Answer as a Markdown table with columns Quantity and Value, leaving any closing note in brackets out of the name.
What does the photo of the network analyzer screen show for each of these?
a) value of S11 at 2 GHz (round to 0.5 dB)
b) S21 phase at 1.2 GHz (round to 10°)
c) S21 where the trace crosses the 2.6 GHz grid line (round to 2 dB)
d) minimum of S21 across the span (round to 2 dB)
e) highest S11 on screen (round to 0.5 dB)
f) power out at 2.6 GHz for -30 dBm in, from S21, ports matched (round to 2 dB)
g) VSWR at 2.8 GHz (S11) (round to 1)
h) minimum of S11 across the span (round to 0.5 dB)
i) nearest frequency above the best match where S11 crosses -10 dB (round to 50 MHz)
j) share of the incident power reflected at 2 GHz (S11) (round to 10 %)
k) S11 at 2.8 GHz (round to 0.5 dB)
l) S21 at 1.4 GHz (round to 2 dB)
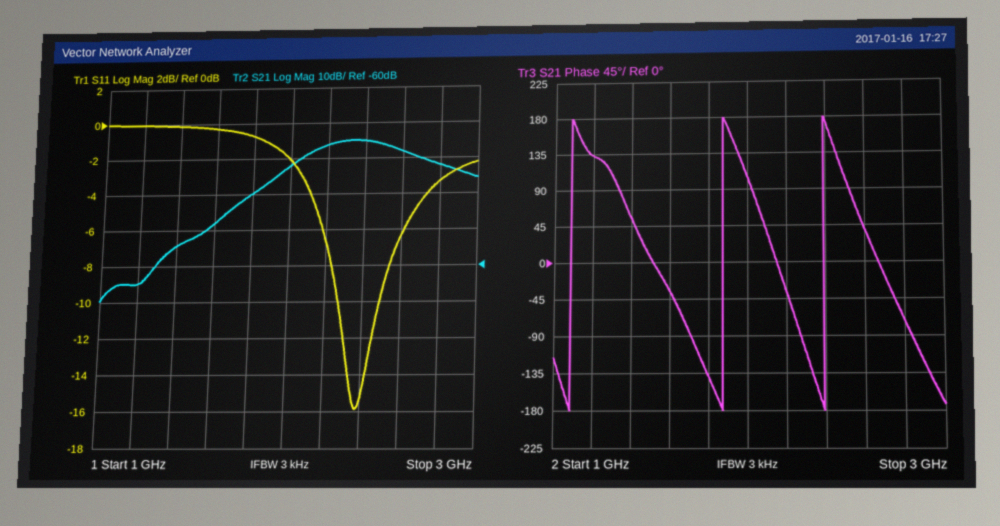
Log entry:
| Quantity | Value |
|---|---|
| value of S11 at 2 GHz | -2.0 dB |
| S21 phase at 1.2 GHz | 130° |
| S21 where the trace crosses the 2.6 GHz grid line | -28 dB |
| minimum of S21 across the span | -70 dB |
| highest S11 on screen | 0.0 dB |
| power out at 2.6 GHz for -30 dBm in, from S21, ports matched | -58 dBm |
| VSWR at 2.8 GHz (S11) | 5 |
| minimum of S11 across the span | -16.0 dB |
| nearest frequency above the best match where S11 crosses -10 dB | 2.50 GHz |
| share of the incident power reflected at 2 GHz (S11) | 60 % |
| S11 at 2.8 GHz | -3.5 dB |
| S21 at 1.4 GHz | -54 dB |
